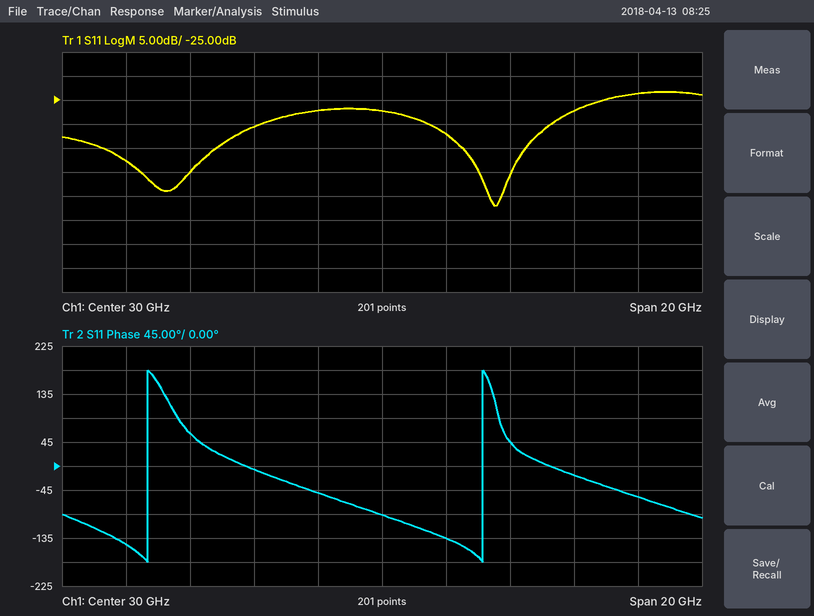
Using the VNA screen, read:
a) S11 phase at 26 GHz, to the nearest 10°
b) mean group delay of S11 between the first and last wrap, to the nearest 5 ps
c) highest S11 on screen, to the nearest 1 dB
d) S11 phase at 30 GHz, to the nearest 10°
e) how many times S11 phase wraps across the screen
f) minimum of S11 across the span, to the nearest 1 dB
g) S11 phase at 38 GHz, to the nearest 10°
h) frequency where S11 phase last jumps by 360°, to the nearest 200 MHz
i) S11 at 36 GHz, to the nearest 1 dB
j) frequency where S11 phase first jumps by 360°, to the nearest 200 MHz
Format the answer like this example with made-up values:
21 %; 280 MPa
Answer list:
-10°; 95 ps; -23 dB; -90°; 2; -47 dB; -60°; 33.2 GHz; -27 dB; 22.6 GHz
